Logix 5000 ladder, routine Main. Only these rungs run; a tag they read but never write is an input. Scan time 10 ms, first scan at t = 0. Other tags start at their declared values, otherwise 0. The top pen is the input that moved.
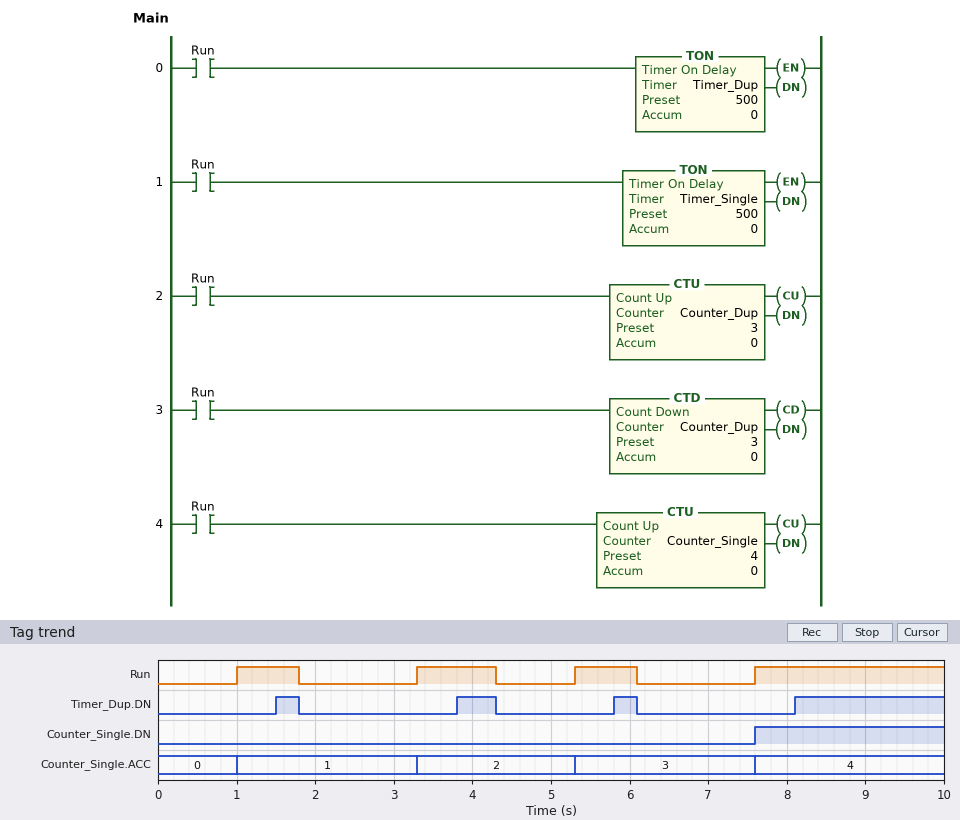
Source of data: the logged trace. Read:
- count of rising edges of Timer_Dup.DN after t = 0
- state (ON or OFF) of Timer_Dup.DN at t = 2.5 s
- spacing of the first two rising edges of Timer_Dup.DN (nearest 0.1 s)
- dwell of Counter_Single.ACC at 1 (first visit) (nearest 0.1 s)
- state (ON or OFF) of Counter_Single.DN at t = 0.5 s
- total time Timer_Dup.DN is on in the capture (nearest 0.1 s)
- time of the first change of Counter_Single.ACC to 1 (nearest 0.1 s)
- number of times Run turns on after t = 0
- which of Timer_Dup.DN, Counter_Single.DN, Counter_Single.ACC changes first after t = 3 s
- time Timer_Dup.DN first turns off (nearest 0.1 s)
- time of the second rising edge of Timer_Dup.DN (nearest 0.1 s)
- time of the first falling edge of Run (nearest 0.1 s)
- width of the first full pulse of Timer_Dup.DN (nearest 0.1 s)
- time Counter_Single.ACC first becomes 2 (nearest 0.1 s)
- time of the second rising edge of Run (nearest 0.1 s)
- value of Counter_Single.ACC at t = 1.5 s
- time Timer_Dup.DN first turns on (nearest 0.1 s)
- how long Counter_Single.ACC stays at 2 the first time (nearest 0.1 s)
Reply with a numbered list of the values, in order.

1. 4
2. OFF
3. 2.3 s
4. 2.3 s
5. OFF
6. 3.0 s
7. 1.0 s
8. 4
9. Counter_Single.ACC
10. 1.8 s
11. 3.8 s
12. 1.8 s
13. 0.3 s
14. 3.3 s
15. 3.3 s
16. 1
17. 1.5 s
18. 2.0 s
